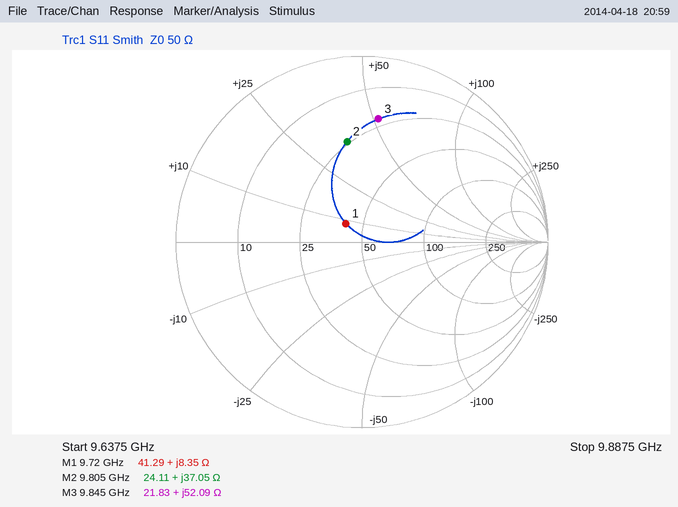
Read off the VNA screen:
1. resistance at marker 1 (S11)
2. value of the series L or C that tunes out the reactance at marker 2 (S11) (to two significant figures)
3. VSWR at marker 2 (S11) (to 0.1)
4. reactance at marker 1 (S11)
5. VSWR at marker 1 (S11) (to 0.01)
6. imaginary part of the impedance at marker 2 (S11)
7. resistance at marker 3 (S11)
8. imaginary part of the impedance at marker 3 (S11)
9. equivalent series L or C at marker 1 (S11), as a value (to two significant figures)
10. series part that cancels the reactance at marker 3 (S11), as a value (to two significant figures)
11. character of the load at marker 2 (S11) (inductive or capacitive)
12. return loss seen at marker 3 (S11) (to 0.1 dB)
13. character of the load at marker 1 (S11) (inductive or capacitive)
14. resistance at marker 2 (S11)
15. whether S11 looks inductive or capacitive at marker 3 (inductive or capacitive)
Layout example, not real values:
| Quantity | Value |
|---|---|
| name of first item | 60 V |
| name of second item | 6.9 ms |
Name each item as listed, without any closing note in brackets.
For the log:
| Quantity | Value |
|---|---|
| resistance at marker 1 | 41.29 Ω |
| value of the series L or C that tunes out the reactance at marker 2 (S11) | 440 fF |
| VSWR at marker 2 (S11) | 3.4 |
| reactance at marker 1 | +8.35 Ω |
| VSWR at marker 1 (S11) | 1.30 |
| imaginary part of the impedance at marker 2 | +37.05 Ω |
| resistance at marker 3 | 21.83 Ω |
| imaginary part of the impedance at marker 3 | +52.09 Ω |
| equivalent series L or C at marker 1 (S11), as a value | 140 pH |
| series part that cancels the reactance at marker 3 (S11), as a value | 310 fF |
| character of the load at marker 2 (S11) | inductive |
| return loss seen at marker 3 (S11) | 3.5 dB |
| character of the load at marker 1 (S11) | inductive |
| resistance at marker 2 | 24.11 Ω |
| whether S11 looks inductive or capacitive at marker 3 | inductive |
